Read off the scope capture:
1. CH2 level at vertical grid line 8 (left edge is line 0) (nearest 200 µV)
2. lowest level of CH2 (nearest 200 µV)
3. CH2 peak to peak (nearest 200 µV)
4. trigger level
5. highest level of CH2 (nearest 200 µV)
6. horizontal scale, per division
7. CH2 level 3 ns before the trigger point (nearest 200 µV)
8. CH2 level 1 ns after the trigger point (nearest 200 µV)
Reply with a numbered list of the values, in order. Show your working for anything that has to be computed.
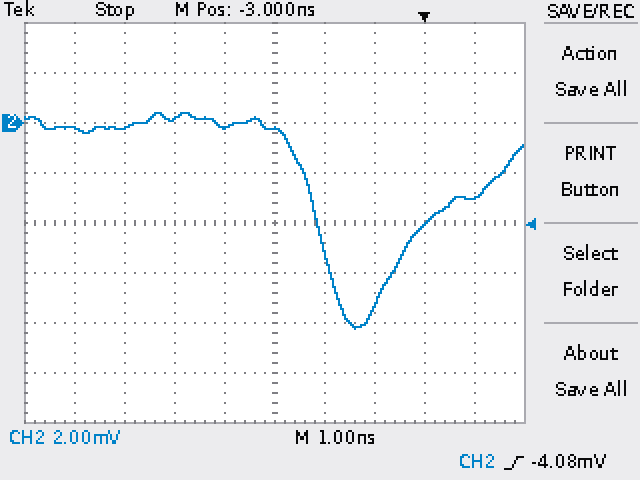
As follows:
1. -4.0 mV
2. -8.2 mV
3. 400 µV − (-8.2 mV) = 8.6 mV
4. -4.08 mV
5. 400 µV
6. 1 ns
7. -200 µV
8. -3.0 mV
